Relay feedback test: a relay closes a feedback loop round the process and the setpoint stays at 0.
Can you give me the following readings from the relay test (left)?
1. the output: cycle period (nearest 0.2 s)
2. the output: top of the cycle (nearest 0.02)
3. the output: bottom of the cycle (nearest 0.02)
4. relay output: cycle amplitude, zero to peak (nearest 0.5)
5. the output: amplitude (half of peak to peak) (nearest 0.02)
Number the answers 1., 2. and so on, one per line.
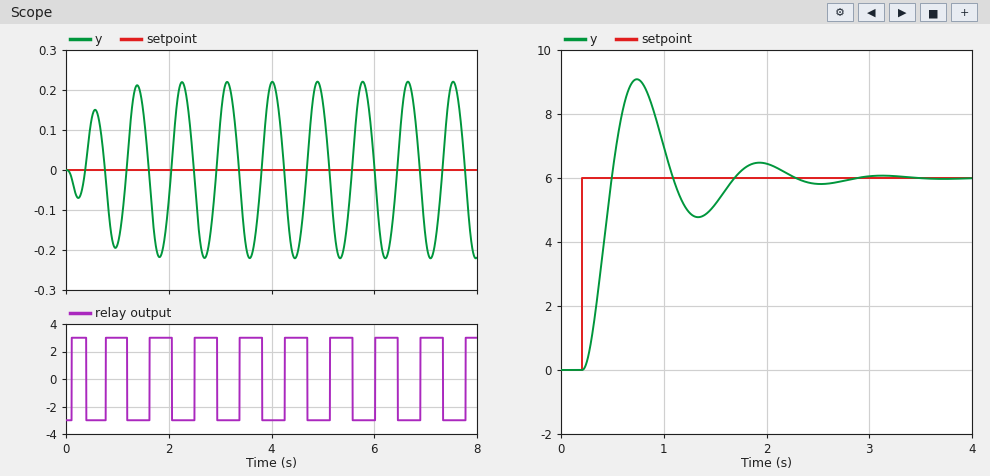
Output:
1. 0.8 s
2. 0.22
3. -0.22
4. 3.0
5. 0.22
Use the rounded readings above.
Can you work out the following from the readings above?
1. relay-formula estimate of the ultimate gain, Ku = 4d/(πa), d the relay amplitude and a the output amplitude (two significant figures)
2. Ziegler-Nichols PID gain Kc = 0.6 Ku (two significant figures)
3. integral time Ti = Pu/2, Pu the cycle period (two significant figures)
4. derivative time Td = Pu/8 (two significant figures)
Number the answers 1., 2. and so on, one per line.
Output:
1. 17
2. 10
3. 0.40 s
4. 0.10 s
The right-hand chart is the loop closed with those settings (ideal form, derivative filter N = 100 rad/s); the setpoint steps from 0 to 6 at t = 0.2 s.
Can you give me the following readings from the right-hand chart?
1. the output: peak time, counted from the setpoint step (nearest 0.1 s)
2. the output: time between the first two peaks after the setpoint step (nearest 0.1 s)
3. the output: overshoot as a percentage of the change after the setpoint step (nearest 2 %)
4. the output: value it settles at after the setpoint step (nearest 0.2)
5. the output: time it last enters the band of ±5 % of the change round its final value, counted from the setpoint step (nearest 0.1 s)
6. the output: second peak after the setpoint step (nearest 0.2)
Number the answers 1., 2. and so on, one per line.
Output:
1. 0.5 s
2. 1.2 s
3. 52 %
4. 6.0
5. 1.9 s
6. 6.4
